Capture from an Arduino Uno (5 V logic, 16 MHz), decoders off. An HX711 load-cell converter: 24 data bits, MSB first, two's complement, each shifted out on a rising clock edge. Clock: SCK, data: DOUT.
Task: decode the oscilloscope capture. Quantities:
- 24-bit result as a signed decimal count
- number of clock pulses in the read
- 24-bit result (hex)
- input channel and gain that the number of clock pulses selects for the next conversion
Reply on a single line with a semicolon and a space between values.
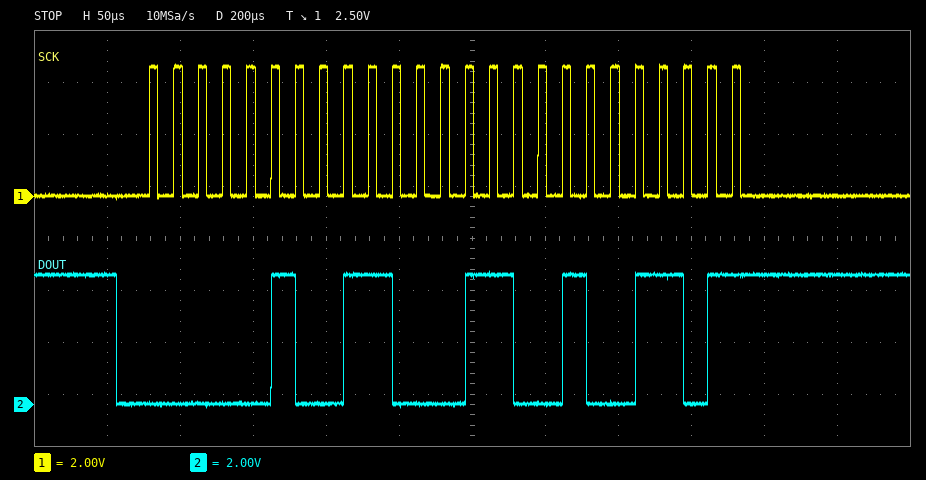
312909; 25; 0x04C64D; channel A, gain 128
